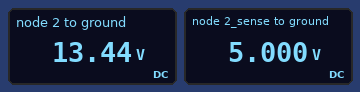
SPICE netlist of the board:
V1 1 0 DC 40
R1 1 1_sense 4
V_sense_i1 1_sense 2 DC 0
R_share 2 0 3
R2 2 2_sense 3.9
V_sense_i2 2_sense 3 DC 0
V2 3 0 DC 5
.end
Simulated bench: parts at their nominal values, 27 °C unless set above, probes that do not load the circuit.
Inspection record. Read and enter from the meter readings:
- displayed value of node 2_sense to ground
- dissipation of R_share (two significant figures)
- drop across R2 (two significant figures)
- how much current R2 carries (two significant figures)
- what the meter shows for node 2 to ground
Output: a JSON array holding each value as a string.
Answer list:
["5.000 V", "60 W", "8.4 V", "2.2 A", "13.44 V"]
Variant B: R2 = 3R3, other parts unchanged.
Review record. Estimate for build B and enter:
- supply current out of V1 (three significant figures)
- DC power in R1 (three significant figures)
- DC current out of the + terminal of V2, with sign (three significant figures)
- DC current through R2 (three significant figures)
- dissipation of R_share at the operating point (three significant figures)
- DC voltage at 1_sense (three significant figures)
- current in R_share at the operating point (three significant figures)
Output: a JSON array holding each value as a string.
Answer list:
["6.75 A", "182 W", "-2.42 A", "2.42 A", "56.3 W", "13.0 V", "4.33 A"]
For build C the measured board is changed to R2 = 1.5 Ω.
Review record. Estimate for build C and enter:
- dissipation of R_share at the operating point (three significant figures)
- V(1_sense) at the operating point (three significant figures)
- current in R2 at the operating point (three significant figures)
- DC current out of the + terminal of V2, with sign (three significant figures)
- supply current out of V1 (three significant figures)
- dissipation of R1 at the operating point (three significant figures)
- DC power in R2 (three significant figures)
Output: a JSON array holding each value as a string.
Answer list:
["37.9 W", "10.7 V", "3.78 A", "-3.78 A", "7.33 A", "215 W", "21.4 W"]
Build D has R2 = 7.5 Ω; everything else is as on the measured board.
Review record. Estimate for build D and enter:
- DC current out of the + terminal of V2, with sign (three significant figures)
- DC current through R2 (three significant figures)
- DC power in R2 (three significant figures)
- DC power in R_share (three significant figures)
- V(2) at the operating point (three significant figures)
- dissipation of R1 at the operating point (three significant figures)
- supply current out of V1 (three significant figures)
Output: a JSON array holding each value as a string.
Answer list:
["-1.32 A", "1.32 A", "13.0 W", "73.8 W", "14.9 V", "158 W", "6.28 A"]
